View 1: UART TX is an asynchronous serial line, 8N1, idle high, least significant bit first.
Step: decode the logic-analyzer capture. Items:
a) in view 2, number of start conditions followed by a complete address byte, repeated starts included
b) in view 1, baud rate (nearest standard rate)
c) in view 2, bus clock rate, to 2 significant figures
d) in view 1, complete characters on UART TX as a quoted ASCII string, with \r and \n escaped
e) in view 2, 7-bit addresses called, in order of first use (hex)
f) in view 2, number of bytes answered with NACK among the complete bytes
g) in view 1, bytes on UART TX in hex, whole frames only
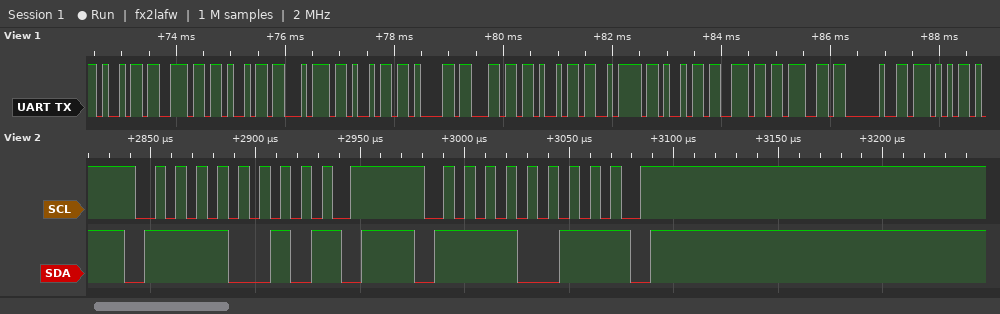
2
9600 baud
100 kHz
"initializing W"
0x79
2
69 6E 69 74 69 61 6C 69 7A 69 6E 67 20 57
